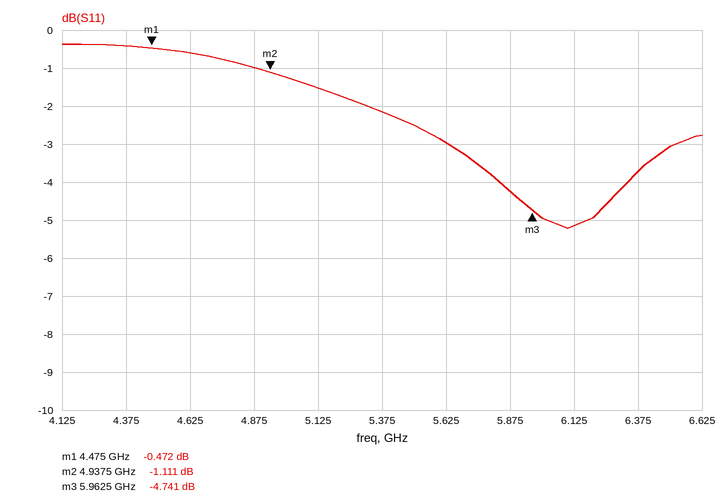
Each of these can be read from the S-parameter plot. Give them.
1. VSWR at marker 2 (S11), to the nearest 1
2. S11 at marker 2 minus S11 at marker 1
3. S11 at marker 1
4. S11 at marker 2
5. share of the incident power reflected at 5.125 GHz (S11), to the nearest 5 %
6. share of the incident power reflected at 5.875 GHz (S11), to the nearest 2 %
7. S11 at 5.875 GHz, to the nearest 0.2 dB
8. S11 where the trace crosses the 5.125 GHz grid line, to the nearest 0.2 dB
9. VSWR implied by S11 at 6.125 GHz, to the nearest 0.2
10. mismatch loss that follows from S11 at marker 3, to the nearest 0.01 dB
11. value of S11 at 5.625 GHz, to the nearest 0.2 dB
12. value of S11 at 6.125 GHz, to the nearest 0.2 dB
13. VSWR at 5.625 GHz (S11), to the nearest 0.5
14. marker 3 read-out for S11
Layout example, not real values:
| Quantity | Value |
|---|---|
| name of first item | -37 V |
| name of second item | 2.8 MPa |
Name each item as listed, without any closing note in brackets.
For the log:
| Quantity | Value |
|---|---|
| VSWR at marker 2 (S11), to the nearest 1 | 16 |
| S11 at marker 2 minus S11 at marker 1 | -0.639 dB |
| S11 at marker 1 | -0.472 dB |
| S11 at marker 2 | -1.111 dB |
| share of the incident power reflected at 5.125 GHz (S11), to the nearest 5 % | 70 % |
| share of the incident power reflected at 5.875 GHz (S11), to the nearest 2 % | 38 % |
| S11 at 5.875 GHz, to the nearest 0.2 dB | -4.2 dB |
| S11 where the trace crosses the 5.125 GHz grid line, to the nearest 0.2 dB | -1.6 dB |
| VSWR implied by S11 at 6.125 GHz, to the nearest 0.2 | 3.4 |
| mismatch loss that follows from S11 at marker 3, to the nearest 0.01 dB | 1.78 dB |
| value of S11 at 5.625 GHz, to the nearest 0.2 dB | -3.0 dB |
| value of S11 at 6.125 GHz, to the nearest 0.2 dB | -5.2 dB |
| VSWR at 5.625 GHz (S11), to the nearest 0.5 | 6.0 |
| marker 3 read-out for S11 | -4.741 dB |
